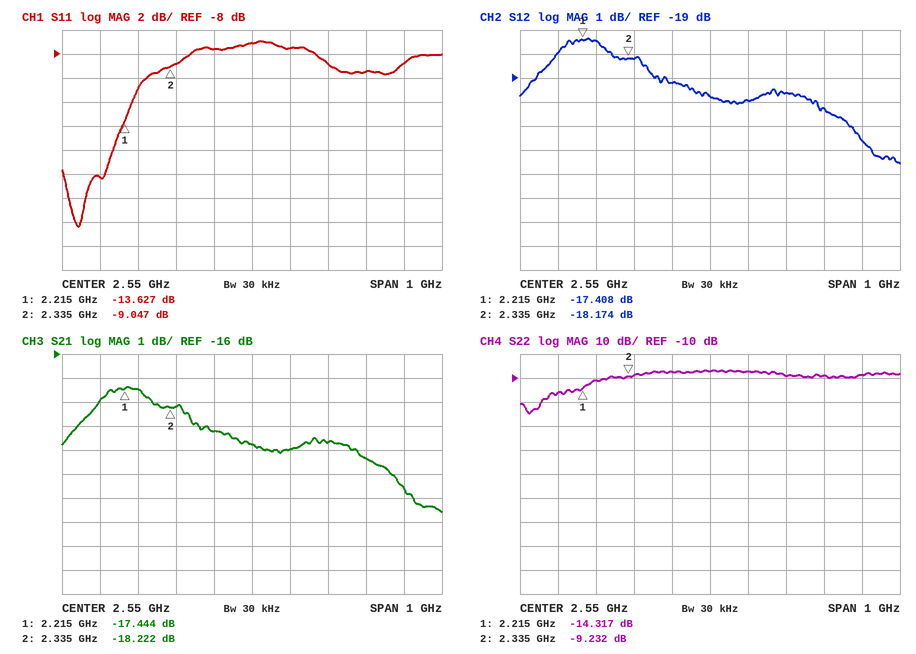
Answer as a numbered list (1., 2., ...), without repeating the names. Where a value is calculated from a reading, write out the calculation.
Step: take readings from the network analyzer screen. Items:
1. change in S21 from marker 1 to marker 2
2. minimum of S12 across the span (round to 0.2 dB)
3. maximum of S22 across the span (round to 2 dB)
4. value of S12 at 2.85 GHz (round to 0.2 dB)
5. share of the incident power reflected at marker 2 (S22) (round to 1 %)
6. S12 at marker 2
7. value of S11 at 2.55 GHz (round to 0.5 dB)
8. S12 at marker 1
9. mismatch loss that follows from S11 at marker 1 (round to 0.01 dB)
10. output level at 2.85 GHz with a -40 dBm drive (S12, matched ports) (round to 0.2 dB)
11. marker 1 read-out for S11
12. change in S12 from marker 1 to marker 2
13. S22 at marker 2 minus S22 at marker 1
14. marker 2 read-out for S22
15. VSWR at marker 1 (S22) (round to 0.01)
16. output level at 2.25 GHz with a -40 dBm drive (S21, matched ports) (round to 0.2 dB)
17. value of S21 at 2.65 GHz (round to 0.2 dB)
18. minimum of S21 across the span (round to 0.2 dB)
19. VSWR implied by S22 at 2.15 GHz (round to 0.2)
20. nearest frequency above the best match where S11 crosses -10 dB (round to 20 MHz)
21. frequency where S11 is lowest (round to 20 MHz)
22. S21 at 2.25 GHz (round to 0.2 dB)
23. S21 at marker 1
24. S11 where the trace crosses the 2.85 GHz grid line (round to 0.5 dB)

1. -18.222 − (-17.444) = -0.778 dB
2. -22.6 dB
3. -6 dB
4. -20.2 dB
5. 10^(-9.232/10) ≈ 12 %
6. -18.174 dB
7. -7.0 dB
8. -17.408 dB
9. −10 log10(1 − 10^(-13.627/10)) ≈ 0.19 dB
10. -40 dBm + (-20.2 dB) = -60.2 dBm
11. -13.627 dB
12. -18.174 − (-17.408) = -0.766 dB
13. -9.232 − (-14.317) = 5.085 dB
14. -9.232 dB
15. (1 + 0.1924)/(1 − 0.1924) ≈ 1.48
16. -40 dBm + (-17.4 dB) = -57.4 dBm
17. -20.0 dB
18. -22.6 dB
19. |Γ| = 10^(-16/20) = 0.1585; VSWR = (1 + 0.1585)/(1 − 0.1585) ≈ 1.4
20. 2.28 GHz
21. 2.10 GHz
22. -17.4 dB
23. -17.444 dB
24. -9.5 dB
